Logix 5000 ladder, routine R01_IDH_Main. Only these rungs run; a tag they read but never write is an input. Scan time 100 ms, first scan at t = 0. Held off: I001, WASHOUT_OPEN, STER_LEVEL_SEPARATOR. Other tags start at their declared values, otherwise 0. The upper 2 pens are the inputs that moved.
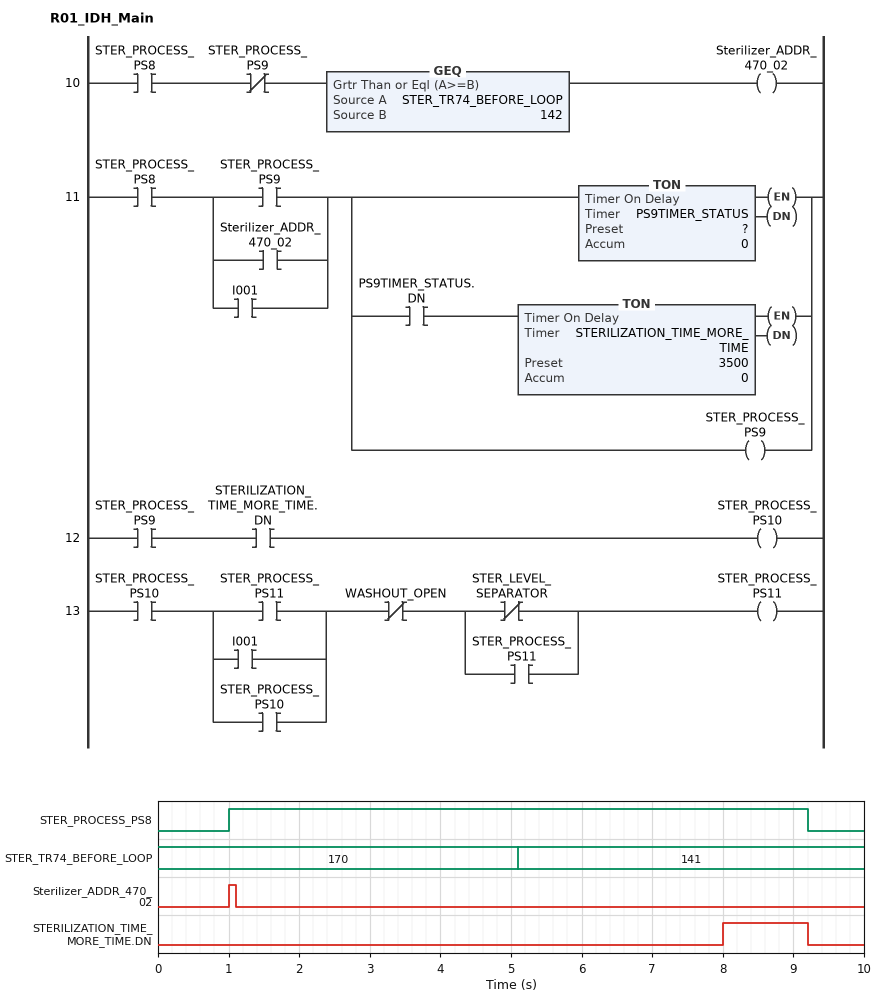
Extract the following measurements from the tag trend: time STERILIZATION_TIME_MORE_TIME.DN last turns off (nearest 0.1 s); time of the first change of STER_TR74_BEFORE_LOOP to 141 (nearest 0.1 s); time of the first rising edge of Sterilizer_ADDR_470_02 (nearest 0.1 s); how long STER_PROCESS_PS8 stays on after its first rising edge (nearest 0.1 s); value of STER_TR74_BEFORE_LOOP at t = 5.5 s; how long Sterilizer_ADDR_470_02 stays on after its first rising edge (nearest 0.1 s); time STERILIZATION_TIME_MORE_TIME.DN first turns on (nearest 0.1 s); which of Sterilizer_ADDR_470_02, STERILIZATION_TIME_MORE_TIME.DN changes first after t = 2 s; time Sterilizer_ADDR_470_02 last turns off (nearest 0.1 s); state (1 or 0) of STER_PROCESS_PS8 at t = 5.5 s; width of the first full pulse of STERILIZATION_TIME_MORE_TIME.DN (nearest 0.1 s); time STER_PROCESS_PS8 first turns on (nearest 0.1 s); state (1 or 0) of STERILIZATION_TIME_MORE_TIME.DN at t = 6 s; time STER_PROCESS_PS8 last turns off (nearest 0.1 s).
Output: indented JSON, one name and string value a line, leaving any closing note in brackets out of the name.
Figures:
{
  "time STERILIZATION_TIME_MORE_TIME.DN last turns off": "9.2 s",
  "time of the first change of STER_TR74_BEFORE_LOOP to 141": "5.1 s",
  "time of the first rising edge of Sterilizer_ADDR_470_02": "1.0 s",
  "how long STER_PROCESS_PS8 stays on after its first rising edge": "8.2 s",
  "value of STER_TR74_BEFORE_LOOP at t = 5.5 s": "141",
  "how long Sterilizer_ADDR_470_02 stays on after its first rising edge": "0.1 s",
  "time STERILIZATION_TIME_MORE_TIME.DN first turns on": "8.0 s",
  "which of Sterilizer_ADDR_470_02, STERILIZATION_TIME_MORE_TIME.DN changes first after t = 2 s": "STERILIZATION_TIME_MORE_TIME.DN",
  "time Sterilizer_ADDR_470_02 last turns off": "1.1 s",
  "state (1 or 0) of STER_PROCESS_PS8 at t = 5.5 s": "1",
  "width of the first full pulse of STERILIZATION_TIME_MORE_TIME.DN": "1.2 s",
  "time STER_PROCESS_PS8 first turns on": "1.0 s",
  "state (1 or 0) of STERILIZATION_TIME_MORE_TIME.DN at t = 6 s": "0",
  "time STER_PROCESS_PS8 last turns off": "9.2 s"
}
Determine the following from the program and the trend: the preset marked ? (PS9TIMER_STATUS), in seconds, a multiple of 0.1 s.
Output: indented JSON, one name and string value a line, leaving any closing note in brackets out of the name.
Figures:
{
  "the preset marked ? (PS9TIMER_STATUS), in seconds, a multiple of 0.1 s": "3.5 s"
}
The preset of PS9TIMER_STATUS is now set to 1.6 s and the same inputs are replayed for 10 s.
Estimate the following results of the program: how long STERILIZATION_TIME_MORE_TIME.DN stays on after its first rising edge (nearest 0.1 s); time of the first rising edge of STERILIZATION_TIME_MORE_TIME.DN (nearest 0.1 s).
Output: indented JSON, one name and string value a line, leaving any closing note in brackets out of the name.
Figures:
{
  "how long STERILIZATION_TIME_MORE_TIME.DN stays on after its first rising edge": "3.1 s",
  "time of the first rising edge of STERILIZATION_TIME_MORE_TIME.DN": "6.1 s"
}
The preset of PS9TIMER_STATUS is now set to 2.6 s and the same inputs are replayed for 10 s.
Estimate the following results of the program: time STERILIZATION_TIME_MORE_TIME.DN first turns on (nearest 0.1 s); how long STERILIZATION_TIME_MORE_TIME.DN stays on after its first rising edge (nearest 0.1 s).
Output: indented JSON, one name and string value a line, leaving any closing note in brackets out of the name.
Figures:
{
  "time STERILIZATION_TIME_MORE_TIME.DN first turns on": "7.1 s",
  "how long STERILIZATION_TIME_MORE_TIME.DN stays on after its first rising edge": "2.1 s"
}
